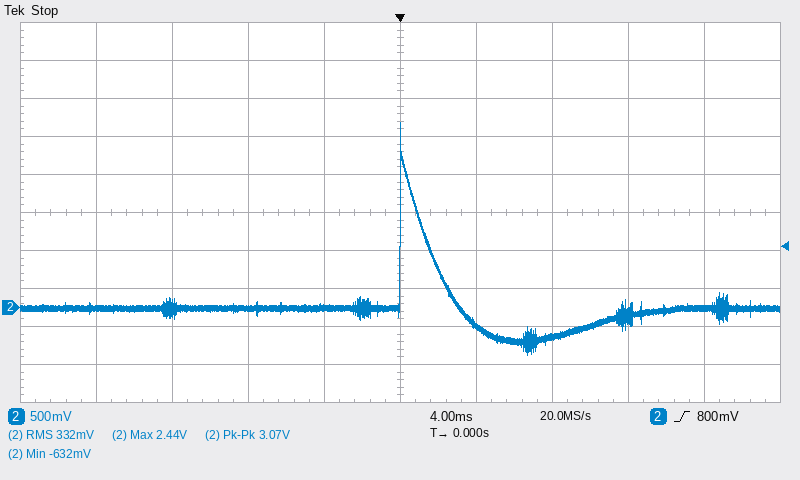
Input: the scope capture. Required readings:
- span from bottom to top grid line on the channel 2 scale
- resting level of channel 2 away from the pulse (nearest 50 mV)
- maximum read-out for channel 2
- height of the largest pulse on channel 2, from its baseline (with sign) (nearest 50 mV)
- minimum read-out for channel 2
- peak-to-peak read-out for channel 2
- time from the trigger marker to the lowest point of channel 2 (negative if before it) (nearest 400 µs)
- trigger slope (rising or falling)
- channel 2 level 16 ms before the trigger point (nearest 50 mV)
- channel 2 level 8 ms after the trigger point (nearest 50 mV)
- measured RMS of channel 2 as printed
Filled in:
5 V
0 mV
2.44 V
+2.45 V
-632 mV
3.07 V
+6.8 ms
rising
0 mV
-400 mV
332 mV
